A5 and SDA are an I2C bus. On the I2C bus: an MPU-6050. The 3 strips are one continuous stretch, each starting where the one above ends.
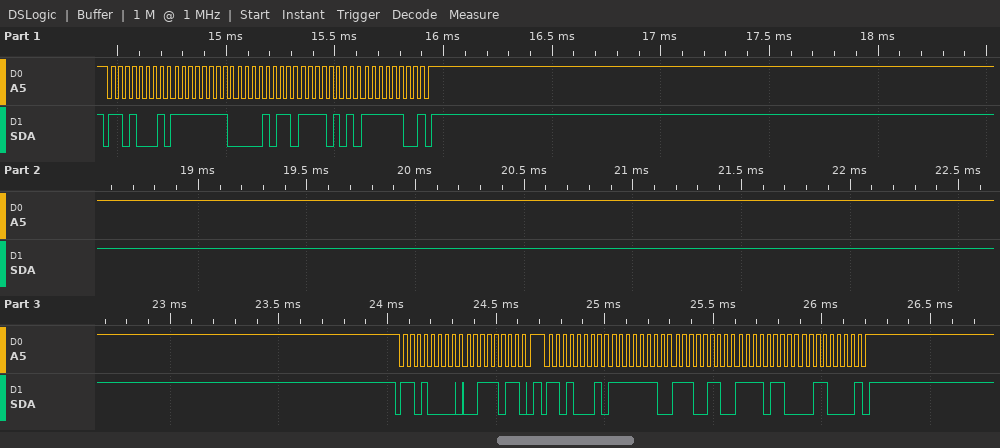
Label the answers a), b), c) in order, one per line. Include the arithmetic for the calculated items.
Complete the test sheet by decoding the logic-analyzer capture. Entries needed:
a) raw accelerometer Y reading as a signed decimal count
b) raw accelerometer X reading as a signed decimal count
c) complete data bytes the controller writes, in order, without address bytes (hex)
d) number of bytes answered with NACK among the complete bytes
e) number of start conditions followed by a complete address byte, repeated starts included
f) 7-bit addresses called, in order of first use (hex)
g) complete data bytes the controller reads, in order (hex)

a) 0xF630 = -2512
b) 0xFEE6 = -282
c) 3B
d) 2
e) 3
f) 0x68
g) FF 0B F5 FC FE E6 F6 30
